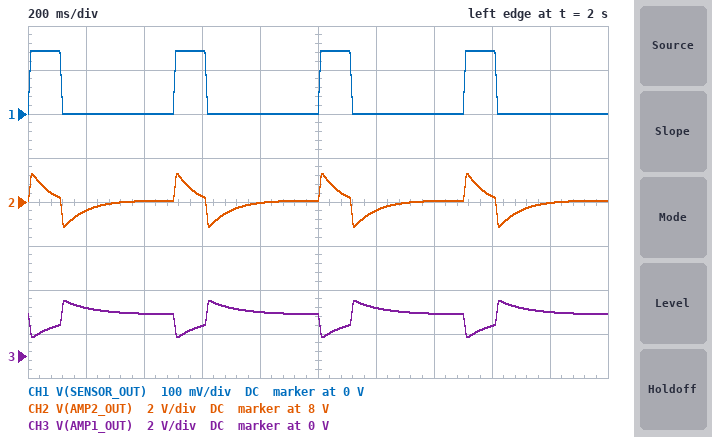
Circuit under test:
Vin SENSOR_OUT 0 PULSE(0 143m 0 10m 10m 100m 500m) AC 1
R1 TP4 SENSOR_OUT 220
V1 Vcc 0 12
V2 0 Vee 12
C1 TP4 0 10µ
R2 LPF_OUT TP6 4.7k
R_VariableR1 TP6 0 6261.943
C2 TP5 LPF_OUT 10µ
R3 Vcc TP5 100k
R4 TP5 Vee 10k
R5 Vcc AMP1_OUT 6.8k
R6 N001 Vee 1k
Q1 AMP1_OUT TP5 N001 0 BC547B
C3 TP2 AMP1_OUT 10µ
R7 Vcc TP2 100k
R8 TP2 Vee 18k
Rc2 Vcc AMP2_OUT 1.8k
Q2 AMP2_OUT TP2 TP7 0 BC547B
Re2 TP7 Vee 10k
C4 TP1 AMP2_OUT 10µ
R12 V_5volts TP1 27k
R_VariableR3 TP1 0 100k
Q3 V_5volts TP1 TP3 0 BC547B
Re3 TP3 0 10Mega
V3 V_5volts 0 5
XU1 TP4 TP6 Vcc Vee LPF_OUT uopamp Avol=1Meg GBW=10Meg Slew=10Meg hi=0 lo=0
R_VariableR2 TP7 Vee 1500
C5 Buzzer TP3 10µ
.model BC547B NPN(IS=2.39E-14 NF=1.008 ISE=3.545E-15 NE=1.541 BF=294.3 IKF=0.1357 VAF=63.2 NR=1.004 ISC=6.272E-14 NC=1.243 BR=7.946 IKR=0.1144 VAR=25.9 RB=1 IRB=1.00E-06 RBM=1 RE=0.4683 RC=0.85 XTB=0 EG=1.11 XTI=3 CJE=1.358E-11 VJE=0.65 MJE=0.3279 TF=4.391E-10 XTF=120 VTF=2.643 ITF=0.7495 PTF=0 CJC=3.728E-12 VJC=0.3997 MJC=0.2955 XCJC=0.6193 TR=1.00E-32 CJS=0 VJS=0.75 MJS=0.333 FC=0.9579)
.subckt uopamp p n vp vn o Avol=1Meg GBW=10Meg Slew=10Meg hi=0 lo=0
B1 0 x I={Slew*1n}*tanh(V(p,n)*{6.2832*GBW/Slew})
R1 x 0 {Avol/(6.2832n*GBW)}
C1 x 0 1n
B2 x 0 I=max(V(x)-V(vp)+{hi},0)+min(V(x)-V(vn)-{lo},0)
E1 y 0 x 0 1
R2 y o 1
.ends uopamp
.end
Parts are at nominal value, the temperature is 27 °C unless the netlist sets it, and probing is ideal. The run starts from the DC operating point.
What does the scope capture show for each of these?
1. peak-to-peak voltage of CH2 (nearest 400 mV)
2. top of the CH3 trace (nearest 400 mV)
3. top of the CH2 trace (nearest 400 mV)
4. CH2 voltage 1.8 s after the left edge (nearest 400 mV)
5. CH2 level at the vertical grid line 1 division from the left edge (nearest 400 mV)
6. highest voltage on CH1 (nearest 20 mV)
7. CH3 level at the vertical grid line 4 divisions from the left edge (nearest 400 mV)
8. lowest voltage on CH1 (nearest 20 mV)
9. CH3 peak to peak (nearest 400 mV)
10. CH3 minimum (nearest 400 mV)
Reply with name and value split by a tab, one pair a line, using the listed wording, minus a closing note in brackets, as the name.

peak-to-peak voltage of CH2	2.4 V
top of the CH3 trace	2.4 V
top of the CH2 trace	9.2 V
CH2 voltage 1.8 s after the left edge	8.0 V
CH2 level at the vertical grid line 1 division from the left edge	7.6 V
highest voltage on CH1	140 mV
CH3 level at the vertical grid line 4 divisions from the left edge	2.0 V
lowest voltage on CH1	0 V
CH3 peak to peak	1.6 V
CH3 minimum	800 mV
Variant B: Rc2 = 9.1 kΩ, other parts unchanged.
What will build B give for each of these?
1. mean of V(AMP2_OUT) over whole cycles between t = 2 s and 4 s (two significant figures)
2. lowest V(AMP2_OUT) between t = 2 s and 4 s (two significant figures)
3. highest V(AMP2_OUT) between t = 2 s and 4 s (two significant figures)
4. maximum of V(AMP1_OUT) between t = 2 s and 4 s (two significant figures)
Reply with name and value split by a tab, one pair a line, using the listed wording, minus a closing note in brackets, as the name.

mean of V(AMP2_OUT) over whole cycles between t = 2 s and 4 s	-7.3 V
lowest V(AMP2_OUT) between t = 2 s and 4 s	-8.8 V
highest V(AMP2_OUT) between t = 2 s and 4 s	-4.5 V
maximum of V(AMP1_OUT) between t = 2 s and 4 s	2.3 V
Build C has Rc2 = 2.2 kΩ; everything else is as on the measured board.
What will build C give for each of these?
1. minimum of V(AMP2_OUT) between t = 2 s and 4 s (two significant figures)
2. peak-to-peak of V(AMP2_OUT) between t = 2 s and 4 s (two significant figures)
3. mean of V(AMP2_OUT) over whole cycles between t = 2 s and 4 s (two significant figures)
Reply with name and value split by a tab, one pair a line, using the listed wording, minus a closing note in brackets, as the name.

minimum of V(AMP2_OUT) between t = 2 s and 4 s	5.8 V
peak-to-peak of V(AMP2_OUT) between t = 2 s and 4 s	2.9 V
mean of V(AMP2_OUT) over whole cycles between t = 2 s and 4 s	7.1 V
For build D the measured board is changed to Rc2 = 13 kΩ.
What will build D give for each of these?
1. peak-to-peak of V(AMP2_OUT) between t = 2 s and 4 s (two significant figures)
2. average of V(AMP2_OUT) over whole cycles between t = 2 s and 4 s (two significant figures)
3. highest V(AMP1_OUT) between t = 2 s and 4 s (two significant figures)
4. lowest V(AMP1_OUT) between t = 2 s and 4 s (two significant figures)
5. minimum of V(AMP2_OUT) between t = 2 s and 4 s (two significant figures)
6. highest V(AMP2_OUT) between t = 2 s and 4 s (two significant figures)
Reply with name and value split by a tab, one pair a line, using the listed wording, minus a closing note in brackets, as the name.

peak-to-peak of V(AMP2_OUT) between t = 2 s and 4 s	2.5 V
average of V(AMP2_OUT) over whole cycles between t = 2 s and 4 s	-9.4 V
highest V(AMP1_OUT) between t = 2 s and 4 s	2.2 V
lowest V(AMP1_OUT) between t = 2 s and 4 s	1.0 V
minimum of V(AMP2_OUT) between t = 2 s and 4 s	-9.7 V
highest V(AMP2_OUT) between t = 2 s and 4 s	-7.2 V
